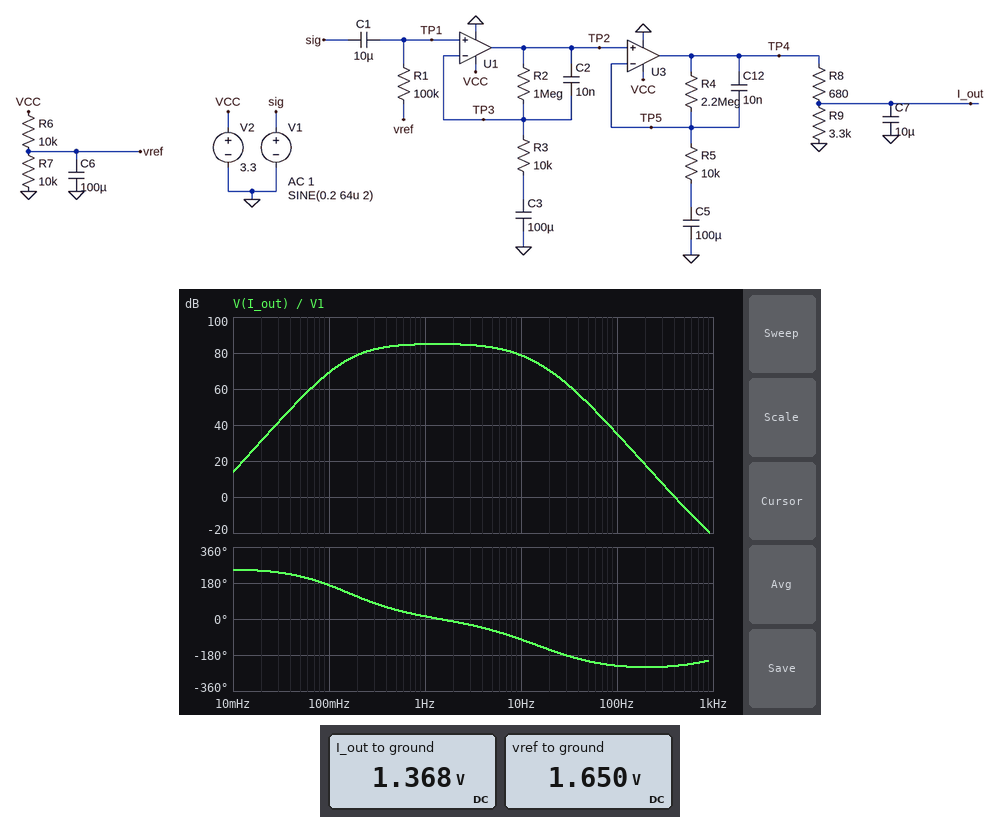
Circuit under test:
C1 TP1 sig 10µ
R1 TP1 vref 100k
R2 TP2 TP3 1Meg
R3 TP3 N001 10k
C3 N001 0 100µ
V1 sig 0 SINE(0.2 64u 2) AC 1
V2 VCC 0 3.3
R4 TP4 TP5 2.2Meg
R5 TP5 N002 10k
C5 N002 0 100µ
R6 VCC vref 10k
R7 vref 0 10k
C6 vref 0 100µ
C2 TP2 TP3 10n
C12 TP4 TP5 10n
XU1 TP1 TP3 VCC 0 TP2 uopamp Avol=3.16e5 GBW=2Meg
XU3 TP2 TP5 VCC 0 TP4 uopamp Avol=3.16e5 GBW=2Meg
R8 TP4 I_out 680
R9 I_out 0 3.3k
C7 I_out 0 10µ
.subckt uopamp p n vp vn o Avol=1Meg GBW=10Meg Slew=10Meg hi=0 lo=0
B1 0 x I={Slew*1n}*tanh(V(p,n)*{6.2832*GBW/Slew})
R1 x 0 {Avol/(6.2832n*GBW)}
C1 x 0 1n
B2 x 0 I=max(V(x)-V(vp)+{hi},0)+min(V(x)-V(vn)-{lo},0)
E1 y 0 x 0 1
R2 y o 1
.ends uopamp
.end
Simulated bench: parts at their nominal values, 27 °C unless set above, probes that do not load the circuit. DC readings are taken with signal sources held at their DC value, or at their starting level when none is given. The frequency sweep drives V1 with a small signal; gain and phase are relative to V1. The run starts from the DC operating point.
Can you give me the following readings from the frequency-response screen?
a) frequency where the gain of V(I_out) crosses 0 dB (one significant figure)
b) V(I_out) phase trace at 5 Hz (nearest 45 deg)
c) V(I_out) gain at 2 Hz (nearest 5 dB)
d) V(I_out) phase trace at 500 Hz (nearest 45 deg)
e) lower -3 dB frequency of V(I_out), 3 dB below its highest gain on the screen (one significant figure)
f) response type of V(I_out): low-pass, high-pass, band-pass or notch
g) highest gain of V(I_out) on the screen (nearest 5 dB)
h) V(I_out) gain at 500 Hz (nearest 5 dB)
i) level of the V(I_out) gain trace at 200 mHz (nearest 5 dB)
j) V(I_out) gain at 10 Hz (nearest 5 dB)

400 Hz
-45 deg
85 dB
-225 deg
300 mHz
band-pass
85 dB
-5 dB
80 dB
80 dB
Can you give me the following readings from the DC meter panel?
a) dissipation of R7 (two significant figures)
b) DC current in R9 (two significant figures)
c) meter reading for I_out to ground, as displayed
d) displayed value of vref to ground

270 µW
410 µA
1.368 V
1.650 V
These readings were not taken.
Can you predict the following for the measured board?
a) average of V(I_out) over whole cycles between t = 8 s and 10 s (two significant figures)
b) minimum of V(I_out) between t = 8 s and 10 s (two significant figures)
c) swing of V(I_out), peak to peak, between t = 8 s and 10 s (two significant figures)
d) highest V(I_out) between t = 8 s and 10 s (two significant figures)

1.4 V
250 mV
2.2 V
2.5 V
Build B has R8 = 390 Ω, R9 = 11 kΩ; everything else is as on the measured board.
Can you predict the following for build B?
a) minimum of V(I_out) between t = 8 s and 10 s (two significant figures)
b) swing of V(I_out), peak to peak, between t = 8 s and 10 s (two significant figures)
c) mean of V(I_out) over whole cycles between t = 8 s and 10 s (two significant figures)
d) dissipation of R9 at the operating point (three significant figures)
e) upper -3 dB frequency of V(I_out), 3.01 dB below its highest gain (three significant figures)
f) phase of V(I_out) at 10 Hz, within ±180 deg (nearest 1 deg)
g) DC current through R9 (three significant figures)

290 mV
2.6 V
1.6 V
231 µW
6.54 Hz
-96 deg
145 µA
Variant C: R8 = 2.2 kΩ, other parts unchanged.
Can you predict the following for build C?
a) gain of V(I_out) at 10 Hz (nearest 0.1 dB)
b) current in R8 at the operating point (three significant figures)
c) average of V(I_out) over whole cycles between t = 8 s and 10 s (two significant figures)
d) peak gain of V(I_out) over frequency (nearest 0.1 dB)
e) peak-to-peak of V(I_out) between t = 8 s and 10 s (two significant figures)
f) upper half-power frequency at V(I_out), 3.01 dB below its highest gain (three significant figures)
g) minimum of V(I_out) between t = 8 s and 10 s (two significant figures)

74.2 dB
300 µA
990 mV
82.1 dB
1.6 V
5.63 Hz
190 mV
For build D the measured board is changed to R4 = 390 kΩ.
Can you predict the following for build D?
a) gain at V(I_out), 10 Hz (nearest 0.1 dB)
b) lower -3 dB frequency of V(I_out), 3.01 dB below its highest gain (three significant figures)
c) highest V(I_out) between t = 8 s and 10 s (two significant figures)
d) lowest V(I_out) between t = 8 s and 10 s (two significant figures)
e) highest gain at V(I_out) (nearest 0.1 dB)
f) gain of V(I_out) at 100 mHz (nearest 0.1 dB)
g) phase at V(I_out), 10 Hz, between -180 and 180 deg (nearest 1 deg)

68.3 dB
304 mHz
1.6 V
1.2 V
70.3 dB
54.3 dB
-62 deg
